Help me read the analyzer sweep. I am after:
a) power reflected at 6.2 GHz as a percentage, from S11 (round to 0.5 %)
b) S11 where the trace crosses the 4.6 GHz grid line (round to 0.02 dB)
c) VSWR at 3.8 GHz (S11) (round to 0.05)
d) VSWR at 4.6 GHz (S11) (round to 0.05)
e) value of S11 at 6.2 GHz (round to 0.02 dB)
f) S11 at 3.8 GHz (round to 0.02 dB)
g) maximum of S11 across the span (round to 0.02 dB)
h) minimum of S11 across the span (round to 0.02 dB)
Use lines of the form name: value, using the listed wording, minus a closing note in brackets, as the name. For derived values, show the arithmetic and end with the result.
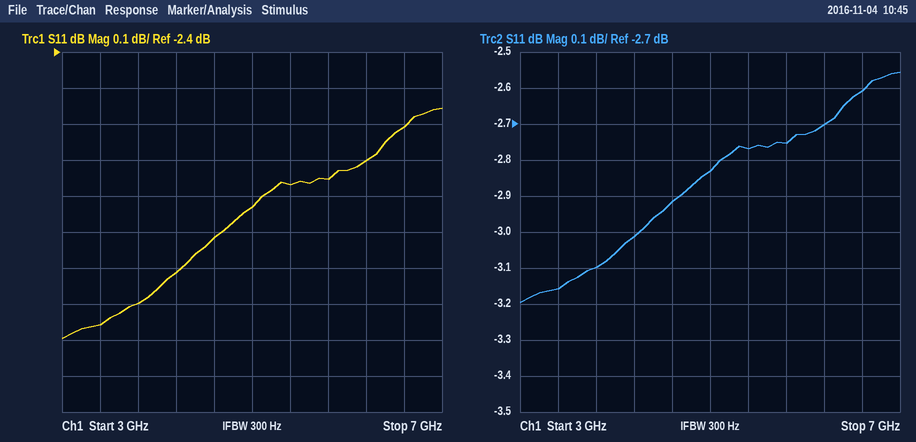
power reflected at 6.2 GHz as a percentage, from S11: 10^(-2.7/10) ≈ 53.7 %, so 53.5 % to the nearest 0.5 %
S11 where the trace crosses the 4.6 GHz grid line: -2.92 dB
VSWR at 3.8 GHz (S11): |Γ| = 10^(-3.1/20) = 0.6998; VSWR = (1 + 0.6998)/(1 − 0.6998) ≈ 5.66, so 5.65 to the nearest 0.05
VSWR at 4.6 GHz (S11): |Γ| = 10^(-2.92/20) = 0.7145; VSWR = (1 + 0.7145)/(1 − 0.7145) ≈ 6.01, so 6.00 to the nearest 0.05
value of S11 at 6.2 GHz: -2.70 dB
S11 at 3.8 GHz: -3.10 dB
maximum of S11 across the span: -2.56 dB
minimum of S11 across the span: -3.20 dB
